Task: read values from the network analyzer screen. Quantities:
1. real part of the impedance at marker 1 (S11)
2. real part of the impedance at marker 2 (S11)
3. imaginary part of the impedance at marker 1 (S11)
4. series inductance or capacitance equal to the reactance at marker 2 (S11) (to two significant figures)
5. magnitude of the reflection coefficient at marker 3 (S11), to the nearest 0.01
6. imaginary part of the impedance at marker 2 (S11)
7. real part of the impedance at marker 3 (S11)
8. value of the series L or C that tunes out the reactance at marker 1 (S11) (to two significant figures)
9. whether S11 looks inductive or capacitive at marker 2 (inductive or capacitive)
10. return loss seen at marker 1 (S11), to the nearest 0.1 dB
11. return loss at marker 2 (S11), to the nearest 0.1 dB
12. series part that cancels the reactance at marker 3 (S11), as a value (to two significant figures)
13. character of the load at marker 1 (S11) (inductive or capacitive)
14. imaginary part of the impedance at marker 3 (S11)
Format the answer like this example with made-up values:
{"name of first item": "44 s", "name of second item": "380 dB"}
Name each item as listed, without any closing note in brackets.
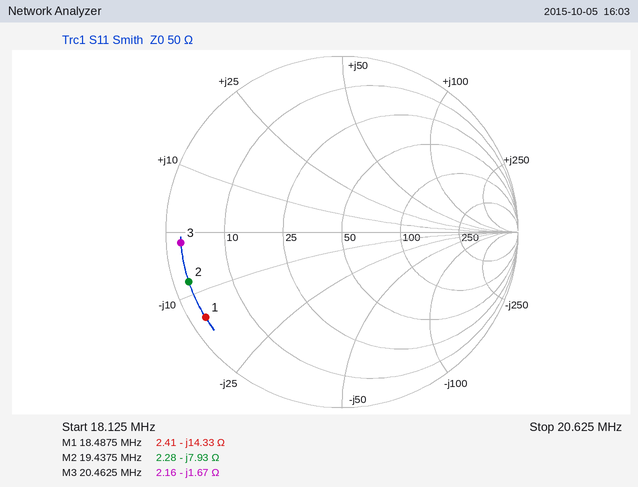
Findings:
{"real part of the impedance at marker 1": "2.41 Ω", "real part of the impedance at marker 2": "2.28 Ω", "imaginary part of the impedance at marker 1": "-14.33 Ω", "series inductance or capacitance equal to the reactance at marker 2 (S11)": "1.0 nF", "magnitude of the reflection coefficient at marker 3 (S11), to the nearest 0.01": "0.92", "imaginary part of the impedance at marker 2": "-7.93 Ω", "real part of the impedance at marker 3": "2.16 Ω", "value of the series L or C that tunes out the reactance at marker 1 (S11)": "120 nH", "whether S11 looks inductive or capacitive at marker 2": "capacitive", "return loss seen at marker 1 (S11), to the nearest 0.1 dB": "0.8 dB", "return loss at marker 2 (S11), to the nearest 0.1 dB": "0.8 dB", "series part that cancels the reactance at marker 3 (S11), as a value": "13 nH", "character of the load at marker 1 (S11)": "capacitive", "imaginary part of the impedance at marker 3": "-1.67 Ω"}
